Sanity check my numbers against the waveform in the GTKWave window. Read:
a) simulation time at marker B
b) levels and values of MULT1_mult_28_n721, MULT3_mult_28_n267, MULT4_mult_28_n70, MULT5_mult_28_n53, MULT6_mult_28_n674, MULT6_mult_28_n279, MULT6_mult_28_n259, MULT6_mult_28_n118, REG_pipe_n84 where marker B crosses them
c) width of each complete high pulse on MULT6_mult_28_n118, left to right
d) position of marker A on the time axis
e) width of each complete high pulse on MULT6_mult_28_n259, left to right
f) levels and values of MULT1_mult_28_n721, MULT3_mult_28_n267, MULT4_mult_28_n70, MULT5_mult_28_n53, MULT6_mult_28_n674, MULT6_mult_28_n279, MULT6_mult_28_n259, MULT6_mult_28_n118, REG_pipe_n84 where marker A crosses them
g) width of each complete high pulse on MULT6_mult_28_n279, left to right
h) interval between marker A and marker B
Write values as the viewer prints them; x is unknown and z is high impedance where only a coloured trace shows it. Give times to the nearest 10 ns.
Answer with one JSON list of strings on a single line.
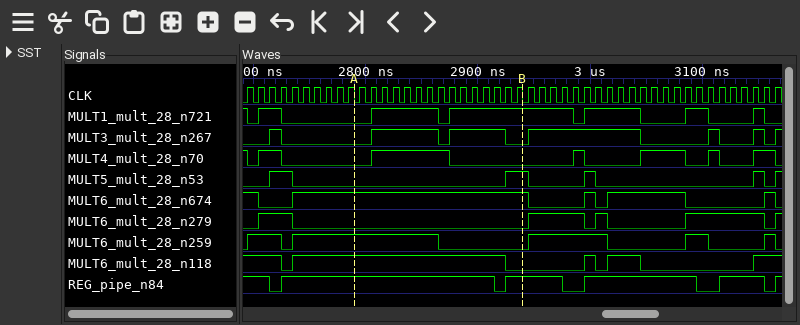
["2940 ns", "MULT1_mult_28_n721=1, MULT3_mult_28_n267=0, MULT4_mult_28_n70=0, MULT5_mult_28_n53=1, MULT6_mult_28_n674=1, MULT6_mult_28_n279=0, MULT6_mult_28_n259=0, MULT6_mult_28_n118=0, REG_pipe_n84=1", "190 ns, 10 ns, 30 ns", "2790 ns", "30 ns, 130 ns, 70 ns, 20 ns, 10 ns", "MULT1_mult_28_n721=0, MULT3_mult_28_n267=0, MULT4_mult_28_n70=0, MULT5_mult_28_n53=0, MULT6_mult_28_n674=1, MULT6_mult_28_n279=0, MULT6_mult_28_n259=1, MULT6_mult_28_n118=1, REG_pipe_n84=1", "30 ns, 50 ns, 10 ns, 70 ns", "150 ns"]
